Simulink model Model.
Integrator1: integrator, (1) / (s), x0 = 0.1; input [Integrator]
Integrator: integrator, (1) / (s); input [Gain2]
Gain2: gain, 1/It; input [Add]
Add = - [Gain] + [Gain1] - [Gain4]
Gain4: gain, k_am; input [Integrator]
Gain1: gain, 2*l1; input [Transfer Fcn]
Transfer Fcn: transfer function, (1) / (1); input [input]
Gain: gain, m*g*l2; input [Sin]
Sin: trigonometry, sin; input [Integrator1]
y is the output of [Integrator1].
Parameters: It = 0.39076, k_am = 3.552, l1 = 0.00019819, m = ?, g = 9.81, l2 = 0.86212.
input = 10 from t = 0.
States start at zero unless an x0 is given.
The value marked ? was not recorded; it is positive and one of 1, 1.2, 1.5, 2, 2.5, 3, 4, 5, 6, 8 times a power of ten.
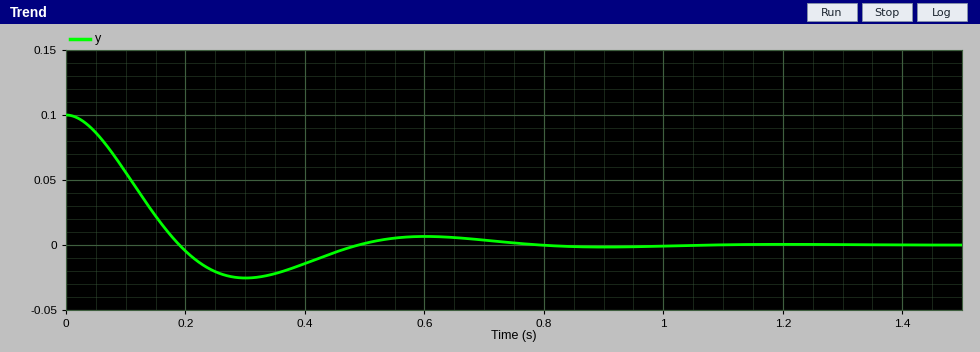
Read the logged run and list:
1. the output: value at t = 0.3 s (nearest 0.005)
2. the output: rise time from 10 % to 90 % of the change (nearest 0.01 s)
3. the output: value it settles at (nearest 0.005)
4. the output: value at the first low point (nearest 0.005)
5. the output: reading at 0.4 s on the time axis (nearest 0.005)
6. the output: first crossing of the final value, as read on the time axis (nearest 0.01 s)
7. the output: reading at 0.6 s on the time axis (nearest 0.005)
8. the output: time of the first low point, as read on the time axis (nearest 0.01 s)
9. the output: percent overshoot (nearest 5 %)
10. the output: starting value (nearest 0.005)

-0.025
0.13 s
0.000
-0.025
-0.015
0.19 s
0.005
0.30 s
25 %
0.100
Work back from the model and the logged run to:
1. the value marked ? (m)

6
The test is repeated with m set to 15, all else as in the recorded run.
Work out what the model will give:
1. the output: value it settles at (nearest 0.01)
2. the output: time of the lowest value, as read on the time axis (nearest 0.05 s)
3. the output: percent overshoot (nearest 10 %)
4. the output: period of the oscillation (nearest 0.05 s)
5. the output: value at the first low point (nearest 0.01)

0.00
0.20 s
40 %
0.35 s
-0.04
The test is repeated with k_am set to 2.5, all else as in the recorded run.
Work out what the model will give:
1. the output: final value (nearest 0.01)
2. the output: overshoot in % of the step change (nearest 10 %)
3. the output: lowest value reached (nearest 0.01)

0.00
40 %
-0.04
